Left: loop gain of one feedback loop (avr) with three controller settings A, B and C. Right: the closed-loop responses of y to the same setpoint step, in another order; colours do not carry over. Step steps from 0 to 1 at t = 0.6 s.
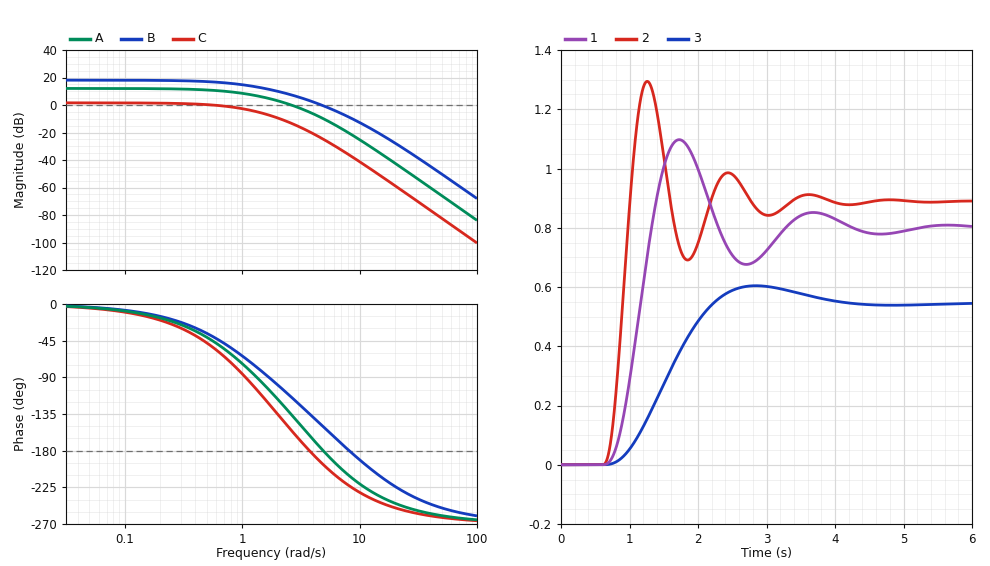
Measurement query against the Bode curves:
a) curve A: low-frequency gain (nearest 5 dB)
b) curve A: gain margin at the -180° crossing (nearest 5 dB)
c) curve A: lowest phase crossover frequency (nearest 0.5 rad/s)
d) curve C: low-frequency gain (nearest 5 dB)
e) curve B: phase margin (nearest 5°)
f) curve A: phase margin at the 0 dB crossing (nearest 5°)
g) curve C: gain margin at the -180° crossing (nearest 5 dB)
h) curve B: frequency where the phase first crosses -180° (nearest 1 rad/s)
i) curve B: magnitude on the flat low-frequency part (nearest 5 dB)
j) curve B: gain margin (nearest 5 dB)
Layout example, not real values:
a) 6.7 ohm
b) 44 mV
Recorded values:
a) 10 dB
b) 10 dB
c) 5.0 rad/s
d) 0 dB
e) 30°
f) 45°
g) 20 dB
h) 8 rad/s
i) 20 dB
j) 10 dB
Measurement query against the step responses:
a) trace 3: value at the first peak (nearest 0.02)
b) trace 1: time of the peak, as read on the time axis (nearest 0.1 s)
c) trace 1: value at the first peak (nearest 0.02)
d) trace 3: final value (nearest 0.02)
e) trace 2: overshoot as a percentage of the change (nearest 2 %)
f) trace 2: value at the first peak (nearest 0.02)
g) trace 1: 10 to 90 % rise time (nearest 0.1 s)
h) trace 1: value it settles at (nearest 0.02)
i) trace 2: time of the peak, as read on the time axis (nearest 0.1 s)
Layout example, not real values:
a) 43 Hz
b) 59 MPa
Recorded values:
a) 0.60
b) 1.7 s
c) 1.10
d) 0.54
e) 46 %
f) 1.30
g) 0.4 s
h) 0.80
i) 1.3 s
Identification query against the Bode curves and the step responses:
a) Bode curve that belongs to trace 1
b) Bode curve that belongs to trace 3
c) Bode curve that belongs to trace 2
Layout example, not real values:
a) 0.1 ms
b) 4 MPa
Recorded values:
a) A
b) C
c) B
